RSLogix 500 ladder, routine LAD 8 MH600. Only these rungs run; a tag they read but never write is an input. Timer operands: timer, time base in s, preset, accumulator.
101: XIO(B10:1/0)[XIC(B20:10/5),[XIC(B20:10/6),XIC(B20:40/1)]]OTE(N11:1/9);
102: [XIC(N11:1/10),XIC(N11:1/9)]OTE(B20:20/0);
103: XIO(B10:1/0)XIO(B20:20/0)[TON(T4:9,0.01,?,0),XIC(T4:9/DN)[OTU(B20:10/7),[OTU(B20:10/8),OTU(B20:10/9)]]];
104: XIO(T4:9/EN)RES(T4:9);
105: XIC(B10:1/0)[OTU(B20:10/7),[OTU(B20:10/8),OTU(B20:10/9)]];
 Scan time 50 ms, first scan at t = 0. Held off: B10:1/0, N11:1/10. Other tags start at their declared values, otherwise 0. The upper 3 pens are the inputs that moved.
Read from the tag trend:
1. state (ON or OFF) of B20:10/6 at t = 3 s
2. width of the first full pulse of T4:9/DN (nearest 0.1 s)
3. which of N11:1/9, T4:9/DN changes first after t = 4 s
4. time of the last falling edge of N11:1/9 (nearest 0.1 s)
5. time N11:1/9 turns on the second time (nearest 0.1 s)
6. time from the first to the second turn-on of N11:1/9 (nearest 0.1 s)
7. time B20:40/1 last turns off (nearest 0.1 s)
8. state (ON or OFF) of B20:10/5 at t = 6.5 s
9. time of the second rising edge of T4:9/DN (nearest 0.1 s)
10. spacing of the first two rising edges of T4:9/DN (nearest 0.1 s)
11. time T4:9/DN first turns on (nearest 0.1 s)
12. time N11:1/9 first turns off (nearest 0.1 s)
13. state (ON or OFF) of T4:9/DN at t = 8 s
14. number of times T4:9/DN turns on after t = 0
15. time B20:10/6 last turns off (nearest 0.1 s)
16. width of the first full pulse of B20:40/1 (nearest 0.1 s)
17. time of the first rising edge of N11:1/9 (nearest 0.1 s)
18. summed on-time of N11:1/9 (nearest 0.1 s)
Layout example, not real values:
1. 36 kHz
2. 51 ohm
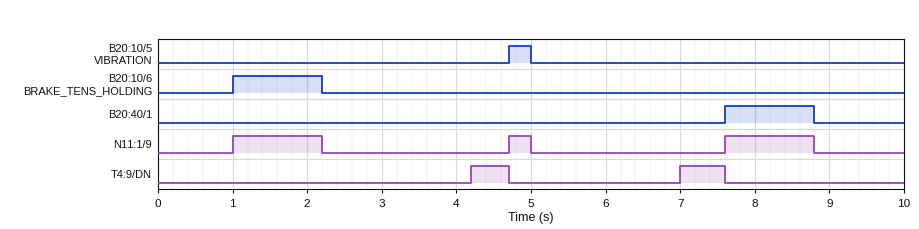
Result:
1. OFF
2. 0.5 s
3. T4:9/DN
4. 8.8 s
5. 4.7 s
6. 3.7 s
7. 8.8 s
8. OFF
9. 7.0 s
10. 2.8 s
11. 4.2 s
12. 2.2 s
13. OFF
14. 2
15. 2.2 s
16. 1.2 s
17. 1.0 s
18. 2.7 s
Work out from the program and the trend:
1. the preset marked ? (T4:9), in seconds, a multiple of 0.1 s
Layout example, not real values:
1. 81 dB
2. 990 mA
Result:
1. 2.0 s
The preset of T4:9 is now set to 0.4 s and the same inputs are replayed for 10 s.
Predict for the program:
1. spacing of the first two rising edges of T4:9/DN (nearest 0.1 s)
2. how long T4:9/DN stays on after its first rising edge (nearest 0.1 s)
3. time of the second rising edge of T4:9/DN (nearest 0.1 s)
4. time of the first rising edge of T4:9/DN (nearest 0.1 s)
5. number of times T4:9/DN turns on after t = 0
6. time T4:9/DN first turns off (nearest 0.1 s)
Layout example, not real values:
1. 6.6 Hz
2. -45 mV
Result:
1. 2.2 s
2. 0.6 s
3. 2.6 s
4. 0.4 s
5. 4
6. 1.0 s
